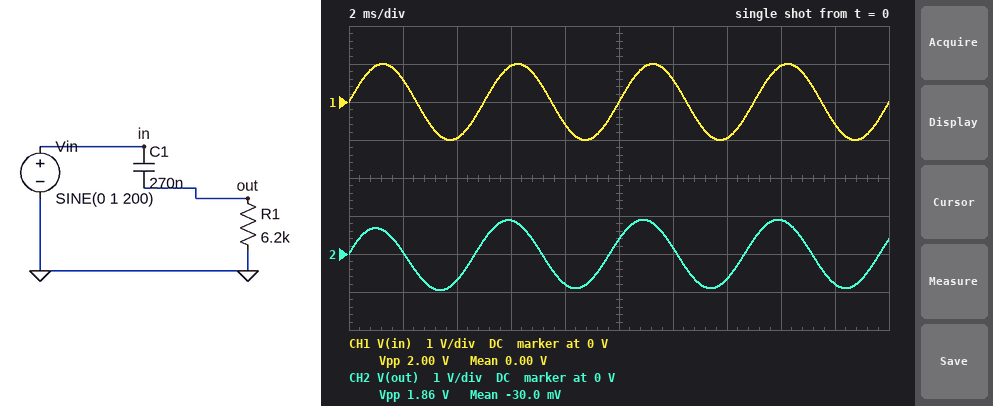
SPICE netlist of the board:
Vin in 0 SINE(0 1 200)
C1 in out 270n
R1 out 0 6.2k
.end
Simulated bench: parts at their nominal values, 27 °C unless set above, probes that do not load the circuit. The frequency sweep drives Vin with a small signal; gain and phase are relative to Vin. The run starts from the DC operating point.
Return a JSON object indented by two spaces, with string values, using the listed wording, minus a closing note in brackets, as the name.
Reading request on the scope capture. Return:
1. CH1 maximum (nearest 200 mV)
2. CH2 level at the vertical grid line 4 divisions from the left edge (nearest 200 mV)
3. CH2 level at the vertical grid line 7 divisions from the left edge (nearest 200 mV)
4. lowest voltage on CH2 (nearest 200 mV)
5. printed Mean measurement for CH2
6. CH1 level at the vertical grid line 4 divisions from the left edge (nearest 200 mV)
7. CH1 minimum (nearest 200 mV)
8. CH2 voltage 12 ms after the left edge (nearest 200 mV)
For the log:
{
  "CH1 maximum": "1.0 V",
  "CH2 level at the vertical grid line 4 divisions from the left edge": "-800 mV",
  "CH2 level at the vertical grid line 7 divisions from the left edge": "-600 mV",
  "lowest voltage on CH2": "-1.0 V",
  "printed Mean measurement for CH2": "-30.0 mV",
  "CH1 level at the vertical grid line 4 divisions from the left edge": "-600 mV",
  "CH1 minimum": "-1.0 V",
  "CH2 voltage 12 ms after the left edge": "200 mV"
}
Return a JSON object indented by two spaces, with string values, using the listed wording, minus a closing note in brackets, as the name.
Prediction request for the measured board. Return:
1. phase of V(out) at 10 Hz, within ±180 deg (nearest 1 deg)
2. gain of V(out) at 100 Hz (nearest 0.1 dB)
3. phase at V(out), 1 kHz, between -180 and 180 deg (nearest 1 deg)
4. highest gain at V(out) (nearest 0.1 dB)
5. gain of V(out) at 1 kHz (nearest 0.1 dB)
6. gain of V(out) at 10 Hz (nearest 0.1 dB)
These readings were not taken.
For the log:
{
  "phase of V(out) at 10 Hz, within ±180 deg": "84 deg",
  "gain of V(out) at 100 Hz": "-2.8 dB",
  "phase at V(out), 1 kHz, between -180 and 180 deg": "5 deg",
  "highest gain at V(out)": "0 dB",
  "gain of V(out) at 1 kHz": "0 dB",
  "gain of V(out) at 10 Hz": "-19.6 dB"
}
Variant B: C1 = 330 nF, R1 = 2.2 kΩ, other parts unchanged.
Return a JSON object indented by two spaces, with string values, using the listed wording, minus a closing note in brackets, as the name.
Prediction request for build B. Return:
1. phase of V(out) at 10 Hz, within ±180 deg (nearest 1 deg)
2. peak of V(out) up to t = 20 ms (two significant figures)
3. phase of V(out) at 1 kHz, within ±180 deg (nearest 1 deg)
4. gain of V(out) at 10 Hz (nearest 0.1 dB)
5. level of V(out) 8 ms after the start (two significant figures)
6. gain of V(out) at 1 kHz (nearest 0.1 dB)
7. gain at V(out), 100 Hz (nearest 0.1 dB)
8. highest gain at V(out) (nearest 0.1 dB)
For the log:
{
  "phase of V(out) at 10 Hz, within ±180 deg": "87 deg",
  "peak of V(out) up to t = 20 ms": "670 mV",
  "phase of V(out) at 1 kHz, within ±180 deg": "12 deg",
  "gain of V(out) at 10 Hz": "-26.8 dB",
  "level of V(out) 8 ms after the start": "-670 mV",
  "gain of V(out) at 1 kHz": "-0.2 dB",
  "gain at V(out), 100 Hz": "-7.6 dB",
  "highest gain at V(out)": "0 dB"
}
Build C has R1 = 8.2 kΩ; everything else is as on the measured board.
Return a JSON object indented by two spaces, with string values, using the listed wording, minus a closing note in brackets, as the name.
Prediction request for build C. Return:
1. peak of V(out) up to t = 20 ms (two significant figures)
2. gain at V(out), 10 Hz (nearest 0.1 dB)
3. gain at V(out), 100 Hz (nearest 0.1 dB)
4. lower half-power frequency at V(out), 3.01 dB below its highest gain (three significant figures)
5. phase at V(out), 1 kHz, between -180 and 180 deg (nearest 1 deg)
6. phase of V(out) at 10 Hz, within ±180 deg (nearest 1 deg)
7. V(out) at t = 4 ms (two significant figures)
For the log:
{
  "peak of V(out) up to t = 20 ms": "940 mV",
  "gain at V(out), 10 Hz": "-17.2 dB",
  "gain at V(out), 100 Hz": "-1.8 dB",
  "lower half-power frequency at V(out), 3.01 dB below its highest gain": "71.9 Hz",
  "phase at V(out), 1 kHz, between -180 and 180 deg": "4 deg",
  "phase of V(out) at 10 Hz, within ±180 deg": "82 deg",
  "V(out) at t = 4 ms": "-800 mV"
}
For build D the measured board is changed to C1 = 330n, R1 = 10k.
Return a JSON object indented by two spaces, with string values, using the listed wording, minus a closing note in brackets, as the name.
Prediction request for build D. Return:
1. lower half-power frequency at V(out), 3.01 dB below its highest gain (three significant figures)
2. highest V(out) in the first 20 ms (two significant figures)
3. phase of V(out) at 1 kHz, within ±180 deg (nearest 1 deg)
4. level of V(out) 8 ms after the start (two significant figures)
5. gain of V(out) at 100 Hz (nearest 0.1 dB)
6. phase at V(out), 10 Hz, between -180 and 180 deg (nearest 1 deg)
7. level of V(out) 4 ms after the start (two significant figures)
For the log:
{
  "lower half-power frequency at V(out), 3.01 dB below its highest gain": "48.2 Hz",
  "highest V(out) in the first 20 ms": "970 mV",
  "phase of V(out) at 1 kHz, within ±180 deg": "3 deg",
  "level of V(out) 8 ms after the start": "-760 mV",
  "gain of V(out) at 100 Hz": "-0.9 dB",
  "phase at V(out), 10 Hz, between -180 and 180 deg": "78 deg",
  "level of V(out) 4 ms after the start": "-900 mV"
}
